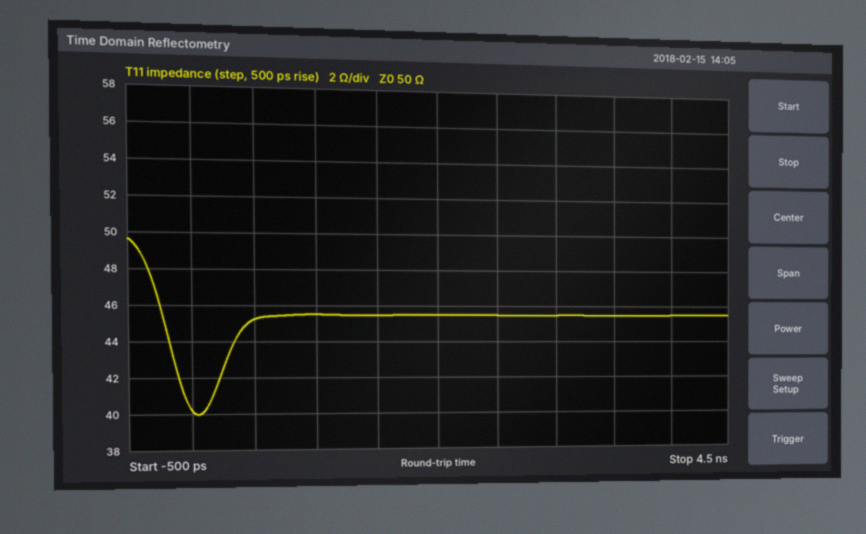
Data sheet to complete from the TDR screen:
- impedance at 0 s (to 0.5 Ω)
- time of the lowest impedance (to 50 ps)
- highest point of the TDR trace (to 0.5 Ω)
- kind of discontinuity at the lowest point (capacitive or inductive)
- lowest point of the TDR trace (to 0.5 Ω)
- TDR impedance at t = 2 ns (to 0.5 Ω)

40.0 Ω
50 ps
49.5 Ω
capacitive
40.0 Ω
45.5 Ω
